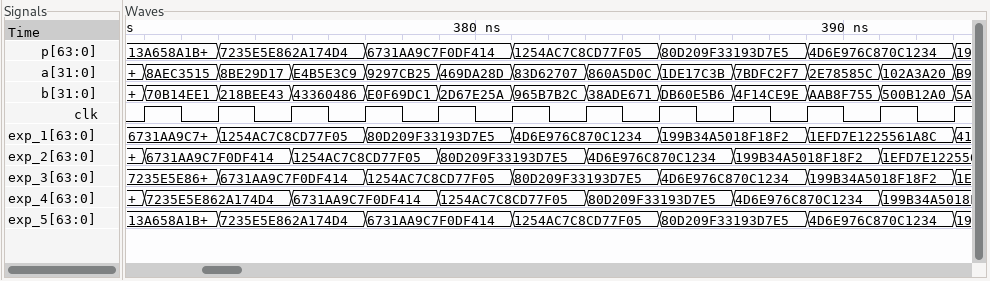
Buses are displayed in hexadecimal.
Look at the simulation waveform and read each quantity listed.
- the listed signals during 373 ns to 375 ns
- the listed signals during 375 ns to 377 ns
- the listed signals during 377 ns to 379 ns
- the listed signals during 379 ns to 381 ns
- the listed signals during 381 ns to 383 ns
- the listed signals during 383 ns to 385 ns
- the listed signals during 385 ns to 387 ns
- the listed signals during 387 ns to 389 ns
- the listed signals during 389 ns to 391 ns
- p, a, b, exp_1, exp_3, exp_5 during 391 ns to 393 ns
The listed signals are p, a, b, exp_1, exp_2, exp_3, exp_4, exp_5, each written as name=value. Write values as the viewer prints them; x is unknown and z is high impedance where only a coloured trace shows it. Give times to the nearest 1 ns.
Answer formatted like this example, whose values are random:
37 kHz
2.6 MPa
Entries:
p=7235E5E862A174D4, a=8BE29D17, b=218BEE43, exp_1=1254AC7C8CD77F05, exp_2=6731AA9C7F0DF414, exp_3=6731AA9C7F0DF414, exp_4=7235E5E862A174D4, exp_5=7235E5E862A174D4
p=7235E5E862A174D4, a=E4B5E3C9, b=43360486, exp_1=1254AC7C8CD77F05, exp_2=1254AC7C8CD77F05, exp_3=6731AA9C7F0DF414, exp_4=6731AA9C7F0DF414, exp_5=7235E5E862A174D4
p=6731AA9C7F0DF414, a=9297CB25, b=E0F69DC1, exp_1=80D209F33193D7E5, exp_2=1254AC7C8CD77F05, exp_3=1254AC7C8CD77F05, exp_4=6731AA9C7F0DF414, exp_5=6731AA9C7F0DF414
p=6731AA9C7F0DF414, a=469DA28D, b=2D67E25A, exp_1=80D209F33193D7E5, exp_2=80D209F33193D7E5, exp_3=1254AC7C8CD77F05, exp_4=1254AC7C8CD77F05, exp_5=6731AA9C7F0DF414
p=1254AC7C8CD77F05, a=83D62707, b=965B7B2C, exp_1=4D6E976C870C1234, exp_2=80D209F33193D7E5, exp_3=80D209F33193D7E5, exp_4=1254AC7C8CD77F05, exp_5=1254AC7C8CD77F05
p=1254AC7C8CD77F05, a=860A5D0C, b=38ADE671, exp_1=4D6E976C870C1234, exp_2=4D6E976C870C1234, exp_3=80D209F33193D7E5, exp_4=80D209F33193D7E5, exp_5=1254AC7C8CD77F05
p=80D209F33193D7E5, a=1DE17C3B, b=DB60E5B6, exp_1=199B34A5018F18F2, exp_2=4D6E976C870C1234, exp_3=4D6E976C870C1234, exp_4=80D209F33193D7E5, exp_5=80D209F33193D7E5
p=80D209F33193D7E5, a=7BDFC2F7, b=4F14CE9E, exp_1=199B34A5018F18F2, exp_2=199B34A5018F18F2, exp_3=4D6E976C870C1234, exp_4=4D6E976C870C1234, exp_5=80D209F33193D7E5
p=4D6E976C870C1234, a=2E78585C, b=AAB8F755, exp_1=1EFD7E1225561A8C, exp_2=199B34A5018F18F2, exp_3=199B34A5018F18F2, exp_4=4D6E976C870C1234, exp_5=4D6E976C870C1234
p=4D6E976C870C1234, a=102A3A20, b=500B12A0, exp_1=1EFD7E1225561A8C, exp_3=199B34A5018F18F2, exp_5=4D6E976C870C1234
